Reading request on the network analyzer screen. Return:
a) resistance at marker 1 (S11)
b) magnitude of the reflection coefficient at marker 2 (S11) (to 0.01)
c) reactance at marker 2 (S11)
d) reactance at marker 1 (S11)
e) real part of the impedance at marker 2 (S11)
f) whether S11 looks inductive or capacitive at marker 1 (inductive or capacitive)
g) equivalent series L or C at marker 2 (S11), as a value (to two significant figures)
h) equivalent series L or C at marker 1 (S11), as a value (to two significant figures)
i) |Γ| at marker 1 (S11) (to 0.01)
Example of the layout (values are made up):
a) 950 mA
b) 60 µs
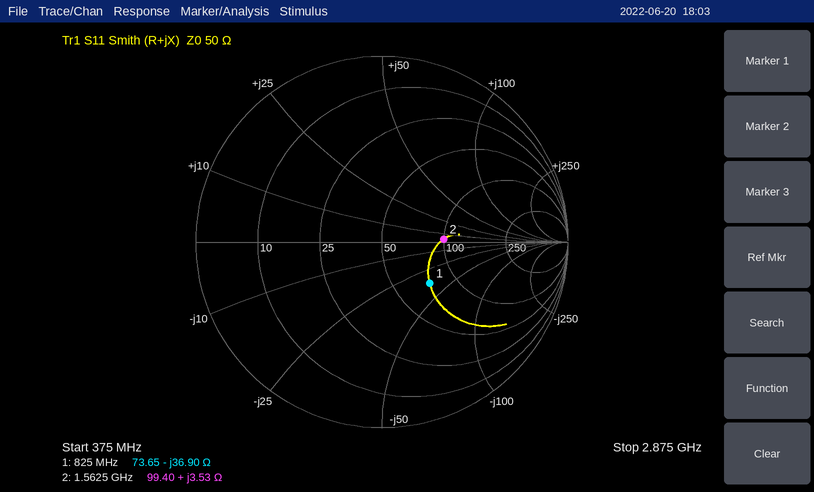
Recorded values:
a) 73.65 Ω
b) 0.33
c) +3.53 Ω
d) -36.90 Ω
e) 99.40 Ω
f) capacitive
g) 360 pH
h) 5.2 pF
i) 0.34
